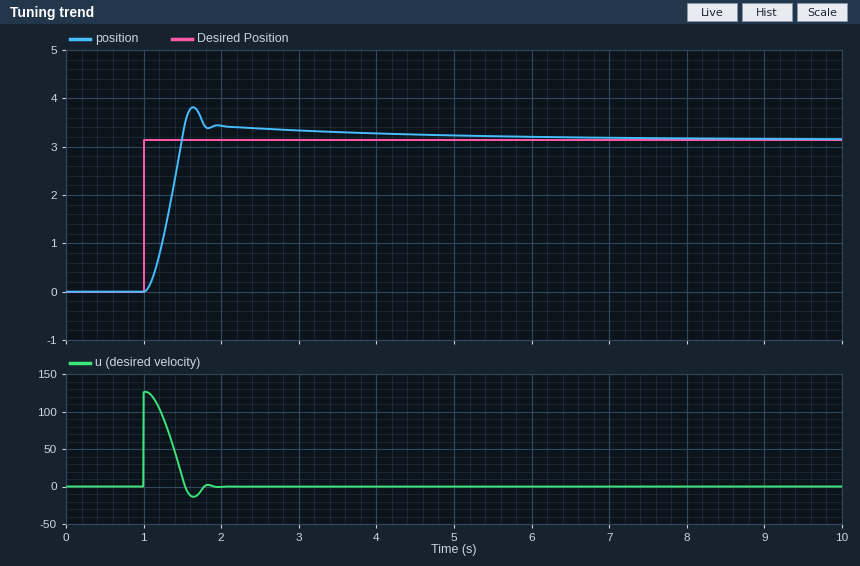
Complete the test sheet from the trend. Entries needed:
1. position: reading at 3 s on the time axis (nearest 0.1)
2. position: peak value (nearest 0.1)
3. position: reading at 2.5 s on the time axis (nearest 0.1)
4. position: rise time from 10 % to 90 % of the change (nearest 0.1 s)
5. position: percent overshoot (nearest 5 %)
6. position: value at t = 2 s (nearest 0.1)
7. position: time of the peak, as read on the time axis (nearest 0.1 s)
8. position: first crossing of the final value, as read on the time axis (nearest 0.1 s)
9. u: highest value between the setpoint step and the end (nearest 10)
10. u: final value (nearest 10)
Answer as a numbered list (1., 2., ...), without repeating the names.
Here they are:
1. 3.3
2. 3.8
3. 3.4
4. 0.3 s
5. 20 %
6. 3.4
7. 1.6 s
8. 1.5 s
9. 130
10. 0
